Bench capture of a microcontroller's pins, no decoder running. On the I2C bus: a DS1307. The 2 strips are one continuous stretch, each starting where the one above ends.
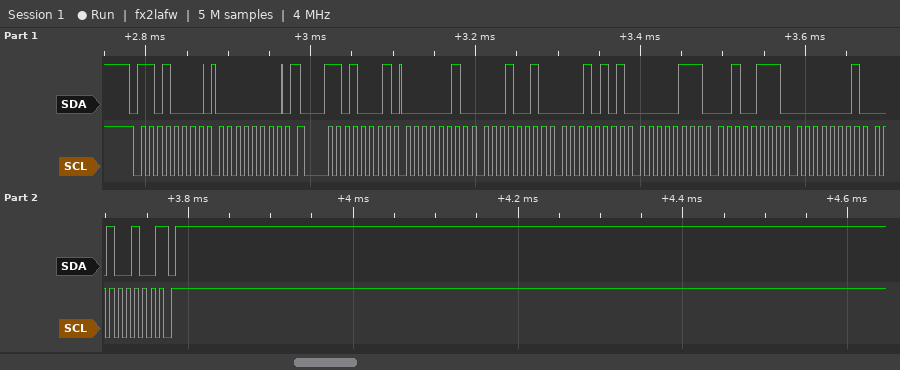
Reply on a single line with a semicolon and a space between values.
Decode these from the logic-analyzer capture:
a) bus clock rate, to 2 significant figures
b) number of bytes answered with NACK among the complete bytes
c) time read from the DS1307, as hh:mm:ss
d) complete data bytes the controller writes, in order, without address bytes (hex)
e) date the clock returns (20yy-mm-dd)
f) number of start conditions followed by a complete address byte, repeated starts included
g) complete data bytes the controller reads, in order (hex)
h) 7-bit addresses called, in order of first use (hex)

100 kHz; 1; 15:12:02; 00; 2024-01-27; 2; 02 12 15 07 27 01 24; 0x68
